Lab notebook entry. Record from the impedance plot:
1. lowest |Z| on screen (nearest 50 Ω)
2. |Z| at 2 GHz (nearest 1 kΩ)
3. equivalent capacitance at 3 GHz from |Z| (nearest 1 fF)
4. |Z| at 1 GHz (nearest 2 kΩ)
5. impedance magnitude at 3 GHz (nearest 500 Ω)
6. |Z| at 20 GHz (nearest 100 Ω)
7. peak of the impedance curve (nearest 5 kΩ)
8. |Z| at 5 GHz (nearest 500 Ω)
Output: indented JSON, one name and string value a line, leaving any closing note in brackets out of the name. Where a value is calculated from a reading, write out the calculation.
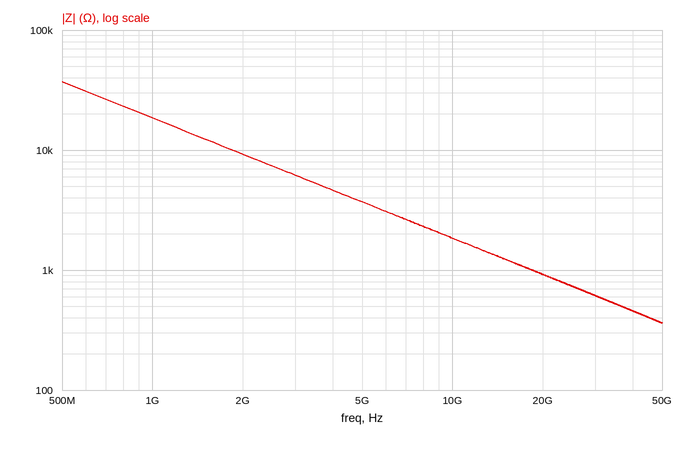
{
  "lowest |Z| on screen": "350 Ω",
  "|Z| at 2 GHz": "9 kΩ",
  "equivalent capacitance at 3 GHz from |Z|": "C = 1/(2π × 3 GHz × 6.0 kΩ) ≈ 9 fF",
  "|Z| at 1 GHz": "18 kΩ",
  "impedance magnitude at 3 GHz": "6.0 kΩ",
  "|Z| at 20 GHz": "900 Ω",
  "peak of the impedance curve": "35 kΩ",
  "|Z| at 5 GHz": "3.5 kΩ"
}
